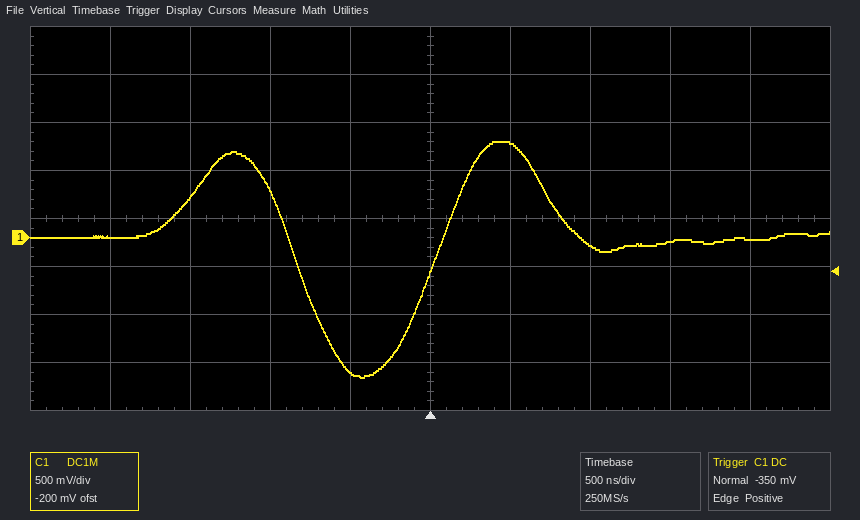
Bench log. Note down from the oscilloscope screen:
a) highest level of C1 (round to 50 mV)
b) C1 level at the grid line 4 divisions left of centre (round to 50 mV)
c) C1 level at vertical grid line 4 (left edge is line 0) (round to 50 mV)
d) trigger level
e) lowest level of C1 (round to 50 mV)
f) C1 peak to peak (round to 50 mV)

1.00 V
0 mV
-1.40 V
-350 mV
-1.45 V
2.45 V
